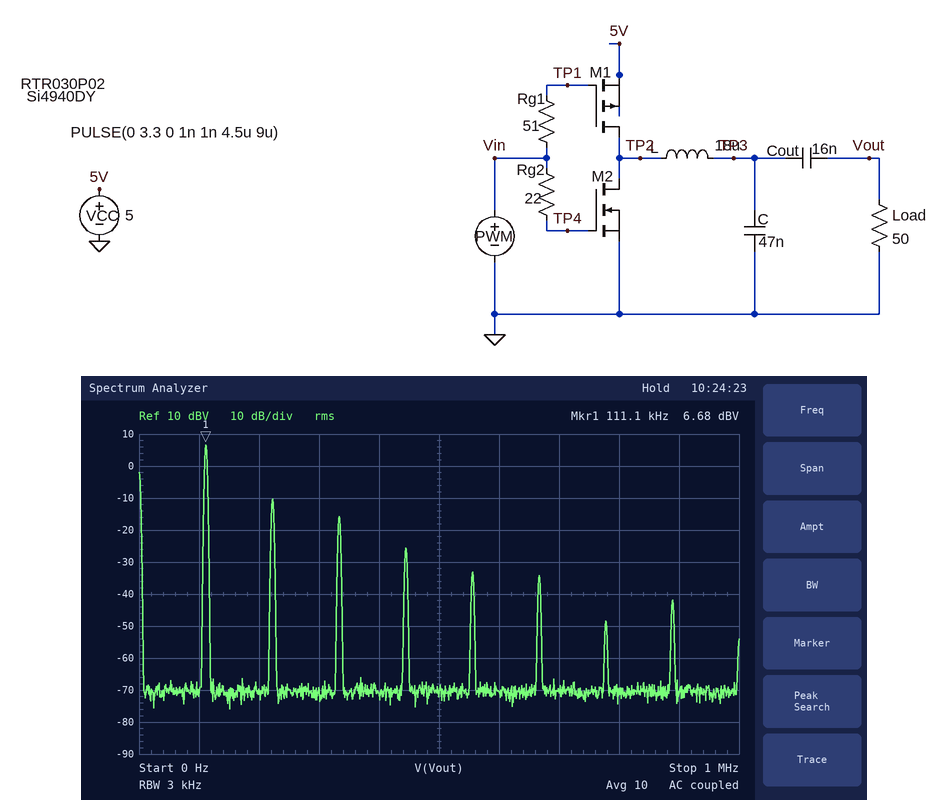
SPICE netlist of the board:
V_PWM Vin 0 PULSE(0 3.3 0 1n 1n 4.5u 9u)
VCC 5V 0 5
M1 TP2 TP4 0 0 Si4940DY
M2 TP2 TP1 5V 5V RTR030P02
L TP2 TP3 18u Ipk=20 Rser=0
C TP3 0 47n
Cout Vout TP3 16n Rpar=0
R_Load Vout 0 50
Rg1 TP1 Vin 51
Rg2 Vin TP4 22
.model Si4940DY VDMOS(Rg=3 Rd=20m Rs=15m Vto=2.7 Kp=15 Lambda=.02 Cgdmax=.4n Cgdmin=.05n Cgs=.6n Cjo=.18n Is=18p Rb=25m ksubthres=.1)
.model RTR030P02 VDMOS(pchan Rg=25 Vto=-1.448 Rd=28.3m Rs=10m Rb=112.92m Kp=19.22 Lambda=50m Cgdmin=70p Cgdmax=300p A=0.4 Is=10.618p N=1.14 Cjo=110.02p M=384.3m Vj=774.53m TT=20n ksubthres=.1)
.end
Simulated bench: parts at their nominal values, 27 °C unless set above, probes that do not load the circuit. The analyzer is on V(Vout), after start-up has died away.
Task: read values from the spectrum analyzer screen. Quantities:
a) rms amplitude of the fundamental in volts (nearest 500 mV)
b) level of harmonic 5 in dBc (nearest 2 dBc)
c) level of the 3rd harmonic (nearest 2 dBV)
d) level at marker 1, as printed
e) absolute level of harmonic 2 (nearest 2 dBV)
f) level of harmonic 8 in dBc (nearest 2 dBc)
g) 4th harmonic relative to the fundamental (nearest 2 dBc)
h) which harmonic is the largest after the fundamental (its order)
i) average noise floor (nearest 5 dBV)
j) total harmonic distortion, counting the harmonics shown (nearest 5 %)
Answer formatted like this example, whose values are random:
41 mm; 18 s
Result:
2.0 V; -40 dBc; -16 dBV; 6.68 dBV; -10 dBV; -48 dBc; -32 dBc; 2; -70 dBV; 15 %
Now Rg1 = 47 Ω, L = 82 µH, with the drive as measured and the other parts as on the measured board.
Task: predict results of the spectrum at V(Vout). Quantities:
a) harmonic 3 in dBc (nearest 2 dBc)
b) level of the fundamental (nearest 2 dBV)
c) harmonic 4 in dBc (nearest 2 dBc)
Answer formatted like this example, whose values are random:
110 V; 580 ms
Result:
-28 dBc; -2 dBV; -38 dBc
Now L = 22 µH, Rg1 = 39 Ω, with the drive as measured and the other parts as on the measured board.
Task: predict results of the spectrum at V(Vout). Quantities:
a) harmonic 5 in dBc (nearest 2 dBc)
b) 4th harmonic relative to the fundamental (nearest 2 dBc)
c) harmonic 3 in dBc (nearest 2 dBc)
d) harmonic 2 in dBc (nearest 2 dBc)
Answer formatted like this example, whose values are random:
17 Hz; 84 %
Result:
-42 dBc; -38 dBc; -26 dBc; -24 dBc
